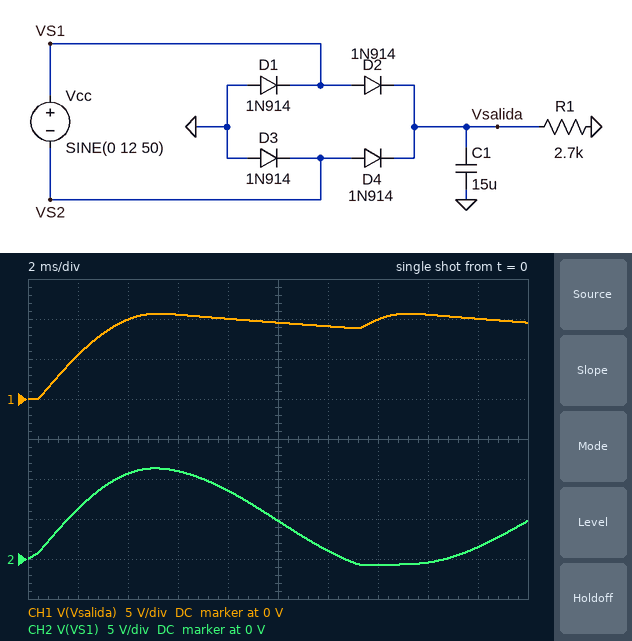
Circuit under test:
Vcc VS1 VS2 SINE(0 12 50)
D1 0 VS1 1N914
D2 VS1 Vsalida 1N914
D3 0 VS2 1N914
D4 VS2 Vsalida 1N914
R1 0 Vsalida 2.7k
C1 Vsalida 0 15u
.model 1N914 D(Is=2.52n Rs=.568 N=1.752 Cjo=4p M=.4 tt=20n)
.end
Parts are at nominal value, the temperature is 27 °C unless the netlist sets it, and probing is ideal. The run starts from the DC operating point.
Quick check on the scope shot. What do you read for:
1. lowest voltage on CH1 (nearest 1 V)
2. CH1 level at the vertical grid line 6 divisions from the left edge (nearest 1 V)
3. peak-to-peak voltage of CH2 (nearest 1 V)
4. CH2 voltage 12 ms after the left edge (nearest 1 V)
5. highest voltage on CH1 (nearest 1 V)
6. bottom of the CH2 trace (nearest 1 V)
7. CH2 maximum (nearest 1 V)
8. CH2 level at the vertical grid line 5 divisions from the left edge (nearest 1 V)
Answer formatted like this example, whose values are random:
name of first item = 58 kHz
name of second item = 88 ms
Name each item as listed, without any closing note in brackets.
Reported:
lowest voltage on CH1 = 0 V
CH1 level at the vertical grid line 6 divisions from the left edge = 9 V
peak-to-peak voltage of CH2 = 12 V
CH2 voltage 12 ms after the left edge = 1 V
highest voltage on CH1 = 11 V
bottom of the CH2 trace = -1 V
CH2 maximum = 11 V
CH2 level at the vertical grid line 5 divisions from the left edge = 5 V
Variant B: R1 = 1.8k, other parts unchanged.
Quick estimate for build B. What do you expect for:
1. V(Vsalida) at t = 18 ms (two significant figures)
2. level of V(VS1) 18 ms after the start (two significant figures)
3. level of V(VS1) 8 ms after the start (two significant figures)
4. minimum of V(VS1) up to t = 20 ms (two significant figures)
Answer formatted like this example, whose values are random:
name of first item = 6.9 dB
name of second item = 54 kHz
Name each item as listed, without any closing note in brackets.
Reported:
V(Vsalida) at t = 18 ms = 9.7 V
level of V(VS1) 18 ms after the start = 1.3 V
level of V(VS1) 8 ms after the start = 8.4 V
minimum of V(VS1) up to t = 20 ms = -770 mV
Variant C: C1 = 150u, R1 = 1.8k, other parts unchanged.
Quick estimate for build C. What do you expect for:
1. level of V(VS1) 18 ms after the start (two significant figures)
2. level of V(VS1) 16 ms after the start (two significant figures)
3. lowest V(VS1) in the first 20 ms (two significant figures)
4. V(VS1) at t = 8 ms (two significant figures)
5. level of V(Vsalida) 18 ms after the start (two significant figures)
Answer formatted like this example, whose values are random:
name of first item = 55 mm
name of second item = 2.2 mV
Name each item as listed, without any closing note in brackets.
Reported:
level of V(VS1) 18 ms after the start = 1.7 V
level of V(VS1) 16 ms after the start = -470 mV
lowest V(VS1) in the first 20 ms = -810 mV
V(VS1) at t = 8 ms = 8.7 V
level of V(Vsalida) 18 ms after the start = 10 V
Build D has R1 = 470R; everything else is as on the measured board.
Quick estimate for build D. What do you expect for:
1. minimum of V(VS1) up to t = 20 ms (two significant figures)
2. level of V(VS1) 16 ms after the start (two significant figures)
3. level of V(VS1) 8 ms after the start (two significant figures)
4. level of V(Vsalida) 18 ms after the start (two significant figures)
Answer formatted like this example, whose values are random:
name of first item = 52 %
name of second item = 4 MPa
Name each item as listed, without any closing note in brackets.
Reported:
minimum of V(VS1) up to t = 20 ms = -800 mV
level of V(VS1) 16 ms after the start = -680 mV
level of V(VS1) 8 ms after the start = 7.4 V
level of V(Vsalida) 18 ms after the start = 7.7 V
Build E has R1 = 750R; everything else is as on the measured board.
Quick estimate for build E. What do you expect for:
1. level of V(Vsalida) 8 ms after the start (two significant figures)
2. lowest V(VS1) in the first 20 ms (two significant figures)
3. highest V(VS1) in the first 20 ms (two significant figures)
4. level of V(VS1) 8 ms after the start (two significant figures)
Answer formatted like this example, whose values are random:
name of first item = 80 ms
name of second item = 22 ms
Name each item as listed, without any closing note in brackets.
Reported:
level of V(Vsalida) 8 ms after the start = 8.5 V
lowest V(VS1) in the first 20 ms = -790 mV
highest V(VS1) in the first 20 ms = 11 V
level of V(VS1) 8 ms after the start = 7.8 V
